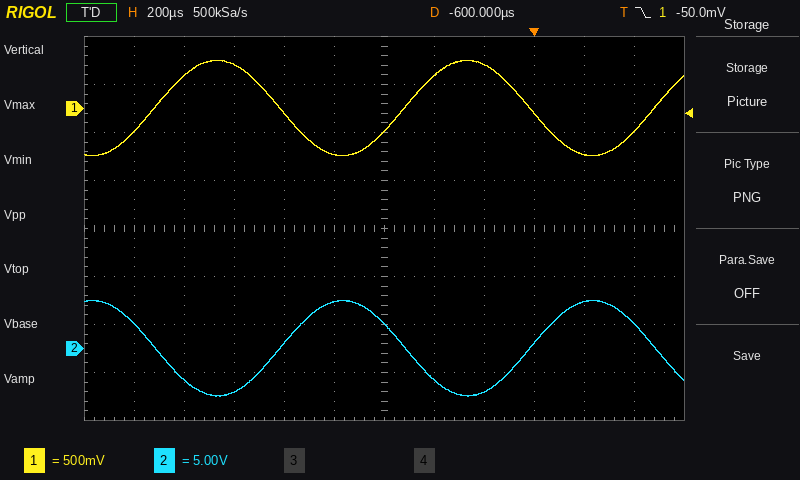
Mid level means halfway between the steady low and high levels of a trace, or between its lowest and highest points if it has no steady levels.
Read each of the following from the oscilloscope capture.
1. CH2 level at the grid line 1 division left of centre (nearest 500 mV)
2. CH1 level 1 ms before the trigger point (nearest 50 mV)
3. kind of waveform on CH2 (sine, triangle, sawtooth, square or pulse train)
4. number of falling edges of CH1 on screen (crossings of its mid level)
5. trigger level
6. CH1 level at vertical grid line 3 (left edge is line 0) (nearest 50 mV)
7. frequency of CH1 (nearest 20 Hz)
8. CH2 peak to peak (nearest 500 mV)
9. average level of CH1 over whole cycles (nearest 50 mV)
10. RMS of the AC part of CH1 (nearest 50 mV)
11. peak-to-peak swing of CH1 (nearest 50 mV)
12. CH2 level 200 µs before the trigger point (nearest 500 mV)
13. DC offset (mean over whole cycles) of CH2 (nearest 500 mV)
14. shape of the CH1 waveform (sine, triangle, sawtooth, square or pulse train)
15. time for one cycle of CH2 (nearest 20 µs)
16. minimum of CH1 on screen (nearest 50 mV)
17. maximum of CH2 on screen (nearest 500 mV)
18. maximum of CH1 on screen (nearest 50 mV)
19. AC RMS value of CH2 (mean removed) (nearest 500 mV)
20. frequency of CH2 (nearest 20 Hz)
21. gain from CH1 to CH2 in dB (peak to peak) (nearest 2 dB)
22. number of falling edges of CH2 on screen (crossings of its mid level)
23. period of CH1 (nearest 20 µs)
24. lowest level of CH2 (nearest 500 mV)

5.0 V
-50 mV
sine
2
-50.0 mV
450 mV
1.00 kHz
10.0 V
0 mV
350 mV
1.00 V
-4.5 V
0.0 V
sine
1.00 ms
-500 mV
5.0 V
500 mV
3.5 V
1.00 kHz
20 dB
3
1.00 ms
-5.0 V
